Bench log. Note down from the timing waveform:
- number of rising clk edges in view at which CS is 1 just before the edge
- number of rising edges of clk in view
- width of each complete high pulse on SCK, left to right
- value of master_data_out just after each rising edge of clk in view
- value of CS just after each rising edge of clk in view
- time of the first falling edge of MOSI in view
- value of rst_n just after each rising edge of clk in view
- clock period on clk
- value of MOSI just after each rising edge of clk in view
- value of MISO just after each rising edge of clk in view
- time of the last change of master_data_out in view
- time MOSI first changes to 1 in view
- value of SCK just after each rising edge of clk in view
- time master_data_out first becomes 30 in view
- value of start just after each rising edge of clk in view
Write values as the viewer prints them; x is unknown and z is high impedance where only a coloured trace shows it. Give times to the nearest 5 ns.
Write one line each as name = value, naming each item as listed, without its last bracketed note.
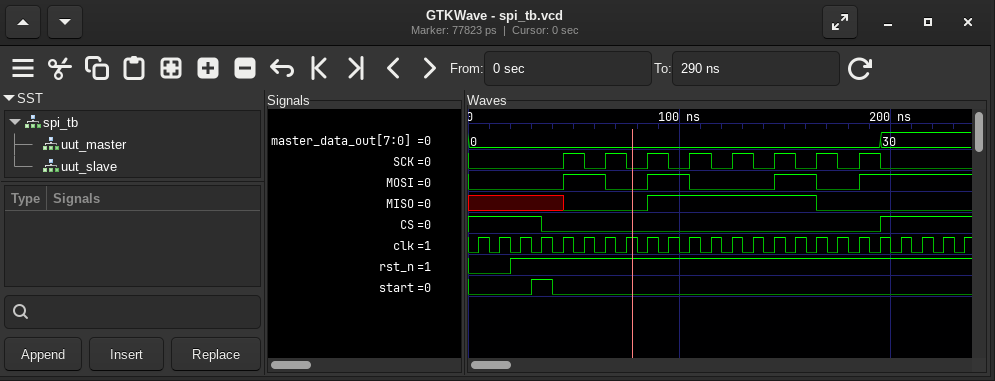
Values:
number of rising clk edges in view at which CS is 1 just before the edge = 8
number of rising edges of clk in view = 24
width of each complete high pulse on SCK, left to right = 10 ns, 10 ns, 10 ns, 10 ns, 10 ns, 10 ns, 10 ns, 10 ns
value of master_data_out just after each rising edge of clk in view = 0, 0, 0, 0, 0, 0, 0, 0, 0, 0, 0, 0, 0, 0, 0, 0, 0, 0, 0, 30, 30, 30, 30, 30
value of CS just after each rising edge of clk in view = 1 1 1 0 0 0 0 0 0 0 0 0 0 0 0 0 0 0 0 1 1 1 1 1
time of the first falling edge of MOSI in view = 65 ns
value of rst_n just after each rising edge of clk in view = 0 0 1 1 1 1 1 1 1 1 1 1 1 1 1 1 1 1 1 1 1 1 1 1
clock period on clk = 10 ns
value of MOSI just after each rising edge of clk in view = 0 0 0 0 1 1 0 0 1 1 0 0 0 0 1 1 0 0 1 1 1 1 1 1
value of MISO just after each rising edge of clk in view = x x x x 0 0 0 0 1 1 1 1 1 1 1 1 0 0 0 0 0 0 0 0
time of the last change of master_data_out in view = 195 ns
time MOSI first changes to 1 in view = 45 ns
value of SCK just after each rising edge of clk in view = 0 0 0 0 1 0 1 0 1 0 1 0 1 0 1 0 1 0 1 0 0 0 0 0
time master_data_out first becomes 30 in view = 195 ns
value of start just after each rising edge of clk in view = 0 0 0 1 0 0 0 0 0 0 0 0 0 0 0 0 0 0 0 0 0 0 0 0
